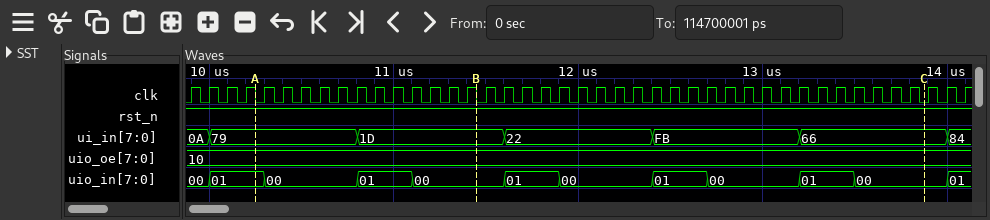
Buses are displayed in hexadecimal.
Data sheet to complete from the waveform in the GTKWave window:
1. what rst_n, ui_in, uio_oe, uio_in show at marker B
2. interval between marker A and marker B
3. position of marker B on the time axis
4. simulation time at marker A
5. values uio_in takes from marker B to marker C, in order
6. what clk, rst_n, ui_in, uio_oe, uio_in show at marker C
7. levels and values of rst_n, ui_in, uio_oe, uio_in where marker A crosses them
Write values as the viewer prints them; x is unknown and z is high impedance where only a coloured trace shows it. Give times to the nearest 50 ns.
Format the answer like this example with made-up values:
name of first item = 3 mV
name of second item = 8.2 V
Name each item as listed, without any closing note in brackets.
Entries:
what rst_n, ui_in, uio_oe, uio_in show at marker B = rst_n=1, ui_in=1D, uio_oe=10, uio_in=00
interval between marker A and marker B = 1200 ns
position of marker B on the time axis = 11450 ns
simulation time at marker A = 10250 ns
values uio_in takes from marker B to marker C, in order = 00, 01, 00, 01, 00, 01, 00
what clk, rst_n, ui_in, uio_oe, uio_in show at marker C = clk=0, rst_n=1, ui_in=66, uio_oe=10, uio_in=00
levels and values of rst_n, ui_in, uio_oe, uio_in where marker A crosses them = rst_n=1, ui_in=79, uio_oe=10, uio_in=01
